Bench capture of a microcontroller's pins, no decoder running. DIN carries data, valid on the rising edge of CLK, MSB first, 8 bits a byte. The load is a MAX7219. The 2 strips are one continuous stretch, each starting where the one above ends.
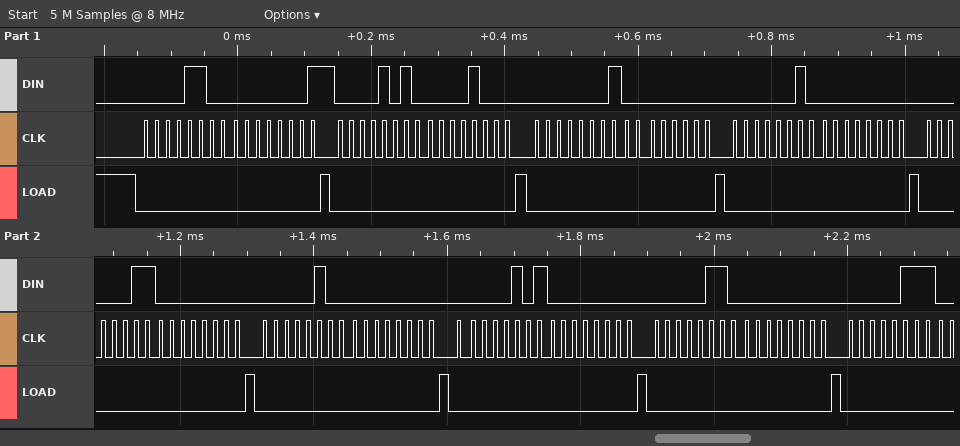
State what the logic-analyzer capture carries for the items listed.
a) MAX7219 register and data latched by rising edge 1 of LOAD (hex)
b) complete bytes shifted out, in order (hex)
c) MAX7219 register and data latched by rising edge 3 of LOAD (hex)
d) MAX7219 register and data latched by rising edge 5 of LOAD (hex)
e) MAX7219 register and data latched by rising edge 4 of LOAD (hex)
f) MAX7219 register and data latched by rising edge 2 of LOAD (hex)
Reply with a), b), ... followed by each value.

a) register 0xC, data 0x01
b) 0C 01 0A 08 01 00 02 00 03 00 04 00 05 00 06 00 07
c) register 0x1, data 0x00
d) register 0x3, data 0x00
e) register 0x2, data 0x00
f) register 0xA, data 0x08
